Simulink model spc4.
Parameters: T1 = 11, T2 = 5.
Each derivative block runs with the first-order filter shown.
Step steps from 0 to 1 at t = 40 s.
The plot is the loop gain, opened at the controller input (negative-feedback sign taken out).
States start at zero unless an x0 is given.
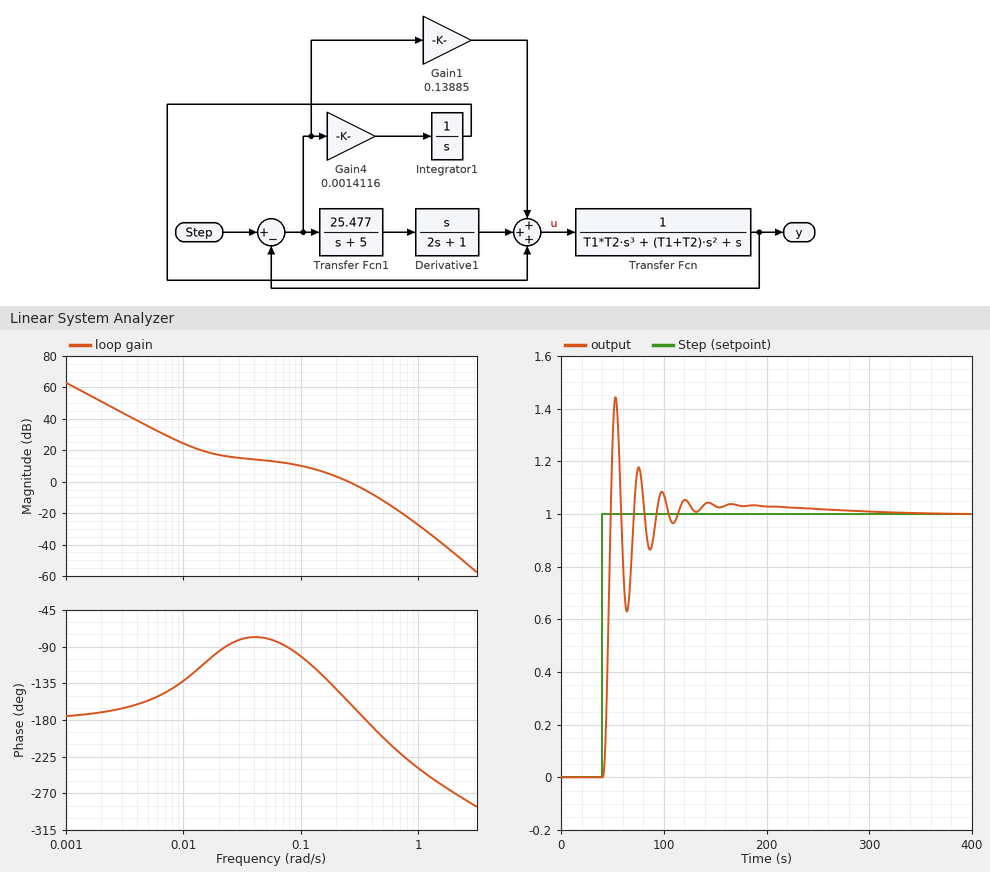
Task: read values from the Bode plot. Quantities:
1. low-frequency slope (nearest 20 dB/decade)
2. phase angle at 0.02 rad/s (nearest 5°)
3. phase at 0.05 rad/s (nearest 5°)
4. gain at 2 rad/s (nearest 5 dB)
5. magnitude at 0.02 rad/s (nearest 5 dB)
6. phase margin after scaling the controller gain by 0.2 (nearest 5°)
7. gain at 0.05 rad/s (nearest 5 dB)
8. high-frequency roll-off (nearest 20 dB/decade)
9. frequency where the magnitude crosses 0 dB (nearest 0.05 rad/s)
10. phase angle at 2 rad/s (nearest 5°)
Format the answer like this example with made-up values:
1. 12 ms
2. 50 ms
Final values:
1. -40 dB/decade
2. -95°
3. -80°
4. -45 dB
5. 15 dB
6. 100°
7. 15 dB
8. -60 dB/decade
9. 0.25 rad/s
10. -270°
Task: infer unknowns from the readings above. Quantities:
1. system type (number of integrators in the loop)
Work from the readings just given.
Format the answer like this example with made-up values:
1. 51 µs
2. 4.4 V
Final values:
1. 2
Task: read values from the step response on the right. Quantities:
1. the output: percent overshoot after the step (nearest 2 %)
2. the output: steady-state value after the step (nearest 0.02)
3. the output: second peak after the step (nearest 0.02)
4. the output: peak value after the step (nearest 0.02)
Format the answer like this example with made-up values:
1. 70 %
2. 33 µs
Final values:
1. 44 %
2. 1.00
3. 1.18
4. 1.44
